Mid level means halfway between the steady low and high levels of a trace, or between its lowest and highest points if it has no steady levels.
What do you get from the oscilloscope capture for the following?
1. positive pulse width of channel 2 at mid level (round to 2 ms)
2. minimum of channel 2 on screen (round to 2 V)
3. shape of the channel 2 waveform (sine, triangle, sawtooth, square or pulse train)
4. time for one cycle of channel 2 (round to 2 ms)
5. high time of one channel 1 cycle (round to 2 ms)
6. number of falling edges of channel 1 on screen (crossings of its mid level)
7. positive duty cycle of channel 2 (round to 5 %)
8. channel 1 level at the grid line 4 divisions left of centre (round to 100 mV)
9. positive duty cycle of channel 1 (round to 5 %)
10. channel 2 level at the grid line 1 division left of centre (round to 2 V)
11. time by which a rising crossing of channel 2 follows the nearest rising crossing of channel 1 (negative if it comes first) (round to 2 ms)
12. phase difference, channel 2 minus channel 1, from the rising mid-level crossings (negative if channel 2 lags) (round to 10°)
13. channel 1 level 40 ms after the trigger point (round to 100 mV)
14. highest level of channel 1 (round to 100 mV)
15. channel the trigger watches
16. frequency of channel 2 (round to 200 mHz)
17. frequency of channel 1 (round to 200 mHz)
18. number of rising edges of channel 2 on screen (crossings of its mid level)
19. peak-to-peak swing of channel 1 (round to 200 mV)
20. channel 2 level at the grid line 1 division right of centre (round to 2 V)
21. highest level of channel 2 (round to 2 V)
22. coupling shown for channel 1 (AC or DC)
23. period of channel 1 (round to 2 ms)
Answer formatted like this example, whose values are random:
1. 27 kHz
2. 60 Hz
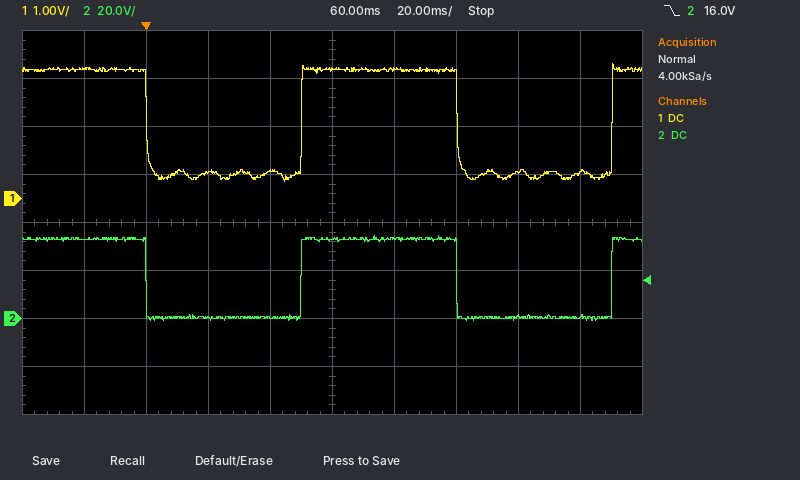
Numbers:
1. 50 ms
2. 0 V
3. square
4. 100 ms
5. 50 ms
6. 2
7. 50 %
8. 2.7 V
9. 50 %
10. 0 V
11. 0 ms
12. 0°
13. 600 mV
14. 2.8 V
15. channel 2
16. 10.0 Hz
17. 10.0 Hz
18. 2
19. 2.4 V
20. 34 V
21. 34 V
22. DC
23. 100 ms
